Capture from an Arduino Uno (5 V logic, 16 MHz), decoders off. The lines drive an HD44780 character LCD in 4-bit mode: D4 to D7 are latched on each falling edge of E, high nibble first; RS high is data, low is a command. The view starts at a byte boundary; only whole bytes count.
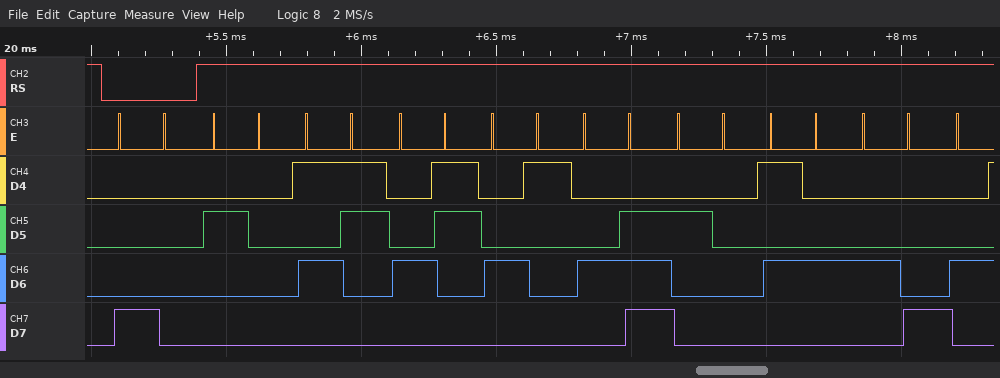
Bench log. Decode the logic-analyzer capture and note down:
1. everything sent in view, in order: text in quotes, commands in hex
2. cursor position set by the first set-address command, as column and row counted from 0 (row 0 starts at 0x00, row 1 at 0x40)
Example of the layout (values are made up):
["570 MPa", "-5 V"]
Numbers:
["0x80 \" SCAN TH\"", "column 0, row 0"]
